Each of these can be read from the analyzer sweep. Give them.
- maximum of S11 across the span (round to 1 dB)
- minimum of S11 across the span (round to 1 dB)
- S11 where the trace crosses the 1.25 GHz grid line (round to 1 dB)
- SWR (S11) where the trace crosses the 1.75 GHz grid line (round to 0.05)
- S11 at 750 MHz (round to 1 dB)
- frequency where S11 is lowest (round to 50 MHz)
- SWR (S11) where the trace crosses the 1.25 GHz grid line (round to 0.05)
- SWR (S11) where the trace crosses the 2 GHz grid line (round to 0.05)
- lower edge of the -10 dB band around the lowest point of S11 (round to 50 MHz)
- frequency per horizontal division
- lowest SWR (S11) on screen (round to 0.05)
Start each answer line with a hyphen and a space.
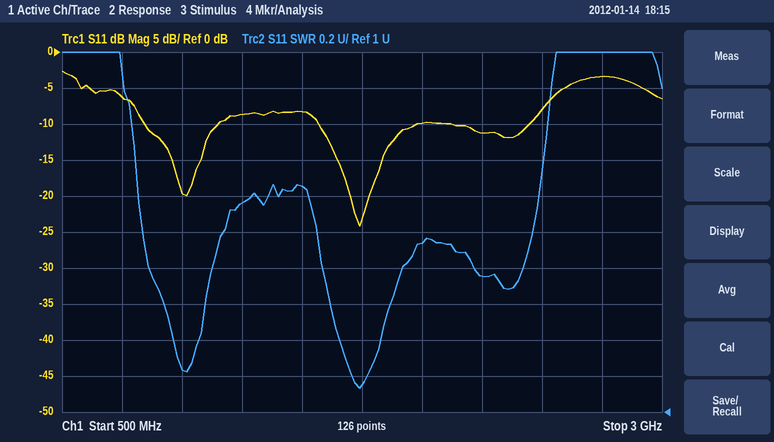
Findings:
- -3 dB
- -24 dB
- -9 dB
- 1.15
- -6 dB
- 1.75 GHz
- 2.15
- 1.95
- 1.55 GHz
- 250 MHz
- 1.15
